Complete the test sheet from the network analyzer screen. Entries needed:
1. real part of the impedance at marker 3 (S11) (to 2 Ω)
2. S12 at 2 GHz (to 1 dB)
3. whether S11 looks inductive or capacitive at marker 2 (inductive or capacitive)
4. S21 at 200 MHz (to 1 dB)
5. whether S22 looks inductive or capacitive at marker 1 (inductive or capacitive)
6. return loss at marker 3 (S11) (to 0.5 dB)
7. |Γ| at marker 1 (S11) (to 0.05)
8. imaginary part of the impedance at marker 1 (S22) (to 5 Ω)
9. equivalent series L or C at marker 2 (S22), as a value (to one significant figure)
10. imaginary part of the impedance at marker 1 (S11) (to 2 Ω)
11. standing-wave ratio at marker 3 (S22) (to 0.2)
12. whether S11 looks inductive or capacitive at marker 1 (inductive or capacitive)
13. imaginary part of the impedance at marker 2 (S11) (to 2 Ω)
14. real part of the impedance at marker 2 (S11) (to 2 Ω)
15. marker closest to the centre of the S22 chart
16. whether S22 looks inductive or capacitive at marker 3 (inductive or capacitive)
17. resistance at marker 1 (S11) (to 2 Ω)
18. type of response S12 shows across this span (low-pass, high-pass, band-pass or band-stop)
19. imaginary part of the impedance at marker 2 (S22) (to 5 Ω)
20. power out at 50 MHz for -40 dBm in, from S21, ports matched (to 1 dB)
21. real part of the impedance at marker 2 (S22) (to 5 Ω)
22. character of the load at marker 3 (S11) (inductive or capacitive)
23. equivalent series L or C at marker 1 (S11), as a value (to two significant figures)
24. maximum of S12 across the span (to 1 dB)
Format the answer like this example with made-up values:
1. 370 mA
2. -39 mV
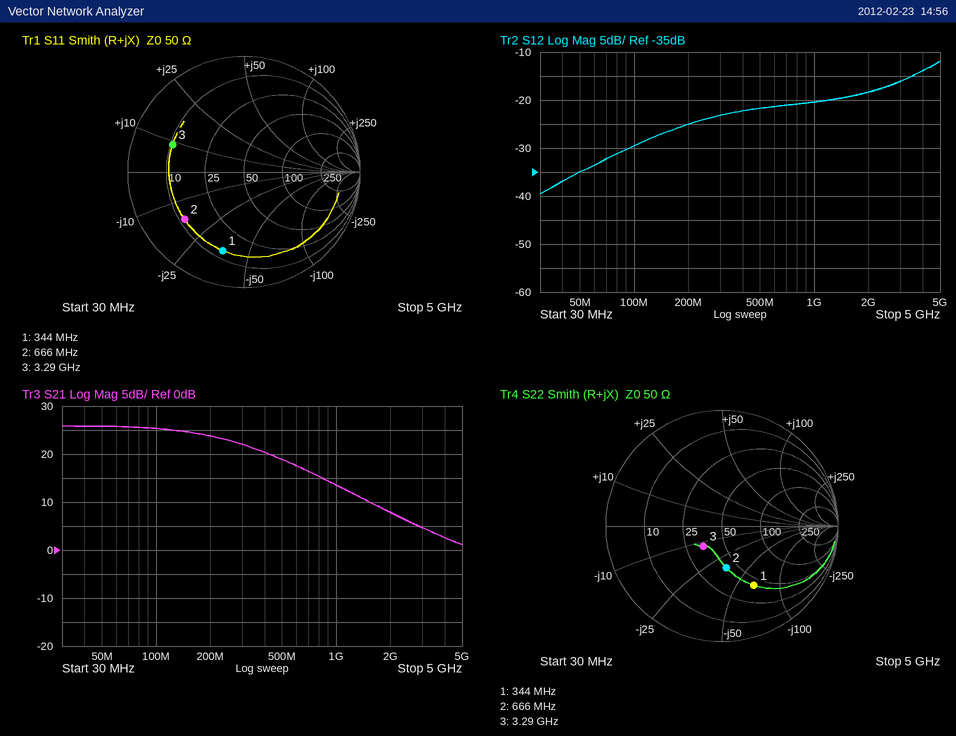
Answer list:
1. 10 Ω
2. -18 dB
3. capacitive
4. 24 dB
5. capacitive
6. 3.5 dB
7. 0.70
8. -65 Ω
9. 7 pF
10. -36 Ω
11. 1.6
12. capacitive
13. -16 Ω
14. 12 Ω
15. marker 3
16. capacitive
17. 14 Ω
18. high-pass
19. -35 Ω
20. -14 dBm
21. 40 Ω
22. inductive
23. 13 pF
24. -12 dB
